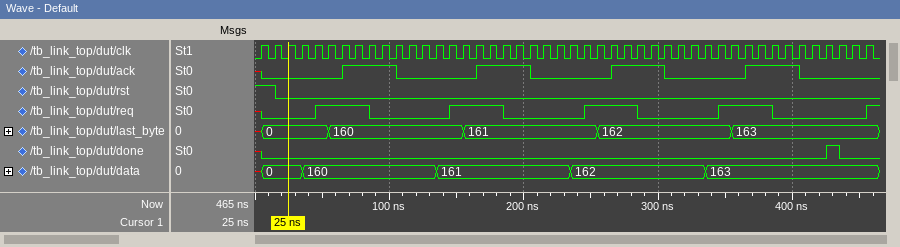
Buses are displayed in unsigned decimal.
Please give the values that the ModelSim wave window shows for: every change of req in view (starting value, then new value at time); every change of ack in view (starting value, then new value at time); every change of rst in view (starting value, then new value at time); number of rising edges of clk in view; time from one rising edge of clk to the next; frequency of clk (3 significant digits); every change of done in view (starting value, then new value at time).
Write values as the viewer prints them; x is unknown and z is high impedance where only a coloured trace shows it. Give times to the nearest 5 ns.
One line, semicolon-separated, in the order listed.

x, 0 at 5 ns, 1 at 45 ns, 0 at 85 ns, 1 at 145 ns, 0 at 185 ns, 1 at 245 ns, 0 at 285 ns, 1 at 345 ns, 0 at 385 ns, 1 at 455 ns; x, 0 at 5 ns, 1 at 65 ns, 0 at 105 ns, 1 at 165 ns, 0 at 205 ns, 1 at 265 ns, 0 at 305 ns, 1 at 365 ns, 0 at 405 ns; 1, 0 at 15 ns; 46; 10 ns; 100 MHz; x, 0 at 5 ns, 1 at 425 ns, 0 at 435 ns
